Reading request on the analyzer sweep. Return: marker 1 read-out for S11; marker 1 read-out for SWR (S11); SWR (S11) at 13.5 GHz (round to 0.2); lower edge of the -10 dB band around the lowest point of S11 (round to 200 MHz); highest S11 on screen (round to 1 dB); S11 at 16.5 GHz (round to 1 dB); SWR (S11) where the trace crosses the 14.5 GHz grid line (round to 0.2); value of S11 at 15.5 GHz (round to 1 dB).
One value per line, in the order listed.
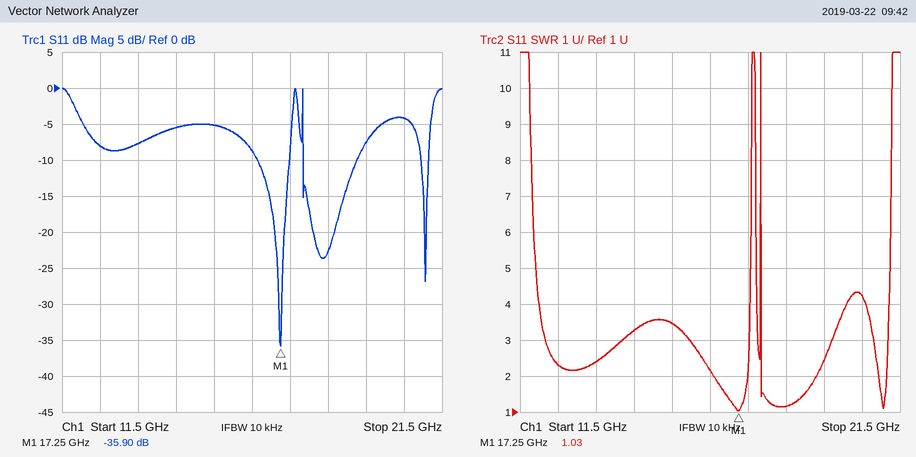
-35.90 dB
1.03
2.4
16.6 GHz
0 dB
-9 dB
3.2
-5 dB
